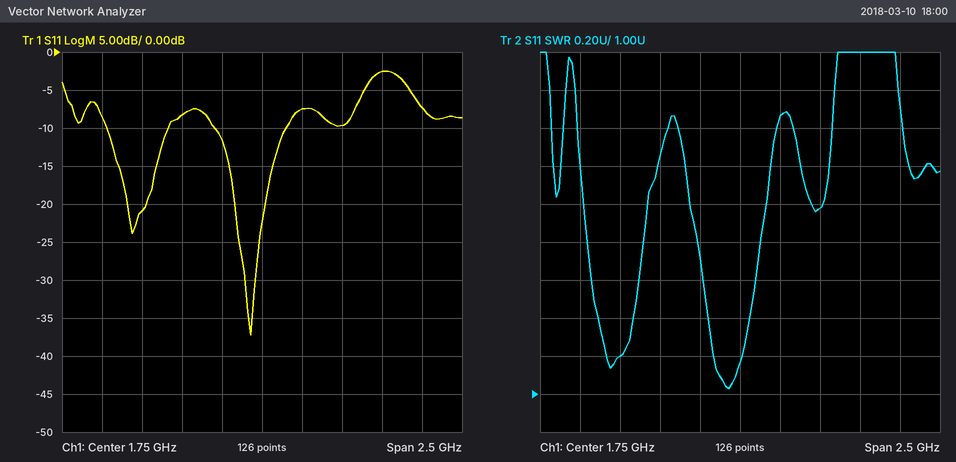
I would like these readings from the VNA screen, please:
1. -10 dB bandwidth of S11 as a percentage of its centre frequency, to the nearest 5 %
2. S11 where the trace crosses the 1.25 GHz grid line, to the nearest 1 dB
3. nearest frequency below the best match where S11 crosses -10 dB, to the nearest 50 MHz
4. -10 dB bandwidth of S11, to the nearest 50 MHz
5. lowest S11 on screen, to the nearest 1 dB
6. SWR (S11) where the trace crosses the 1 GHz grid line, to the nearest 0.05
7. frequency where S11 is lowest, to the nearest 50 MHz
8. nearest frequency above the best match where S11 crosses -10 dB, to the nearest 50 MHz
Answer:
25 %
-8 dB
1.45 GHz
450 MHz
-37 dB
1.20
1.70 GHz
1.90 GHz
